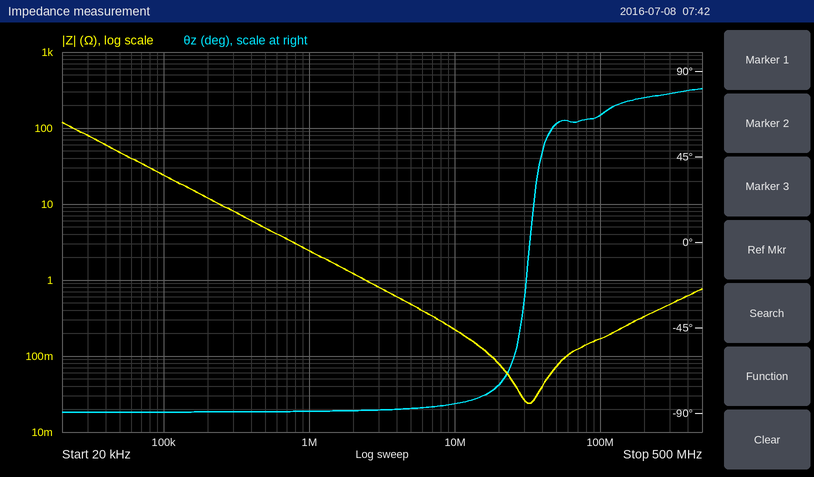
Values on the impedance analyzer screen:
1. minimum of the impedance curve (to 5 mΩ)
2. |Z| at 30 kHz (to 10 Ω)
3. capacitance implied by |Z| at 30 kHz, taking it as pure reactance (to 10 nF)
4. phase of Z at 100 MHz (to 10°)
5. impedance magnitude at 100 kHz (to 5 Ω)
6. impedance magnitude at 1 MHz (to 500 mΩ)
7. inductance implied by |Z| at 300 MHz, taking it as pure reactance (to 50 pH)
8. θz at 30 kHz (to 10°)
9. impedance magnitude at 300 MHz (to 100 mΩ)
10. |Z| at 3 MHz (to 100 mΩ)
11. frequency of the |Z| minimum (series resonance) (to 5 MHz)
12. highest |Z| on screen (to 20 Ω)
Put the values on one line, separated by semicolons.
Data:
25 mΩ; 80 Ω; 70 nF; 70°; 25 Ω; 2.5 Ω; 250 pH; -90°; 500 mΩ; 800 mΩ; 30 MHz; 120 Ω
